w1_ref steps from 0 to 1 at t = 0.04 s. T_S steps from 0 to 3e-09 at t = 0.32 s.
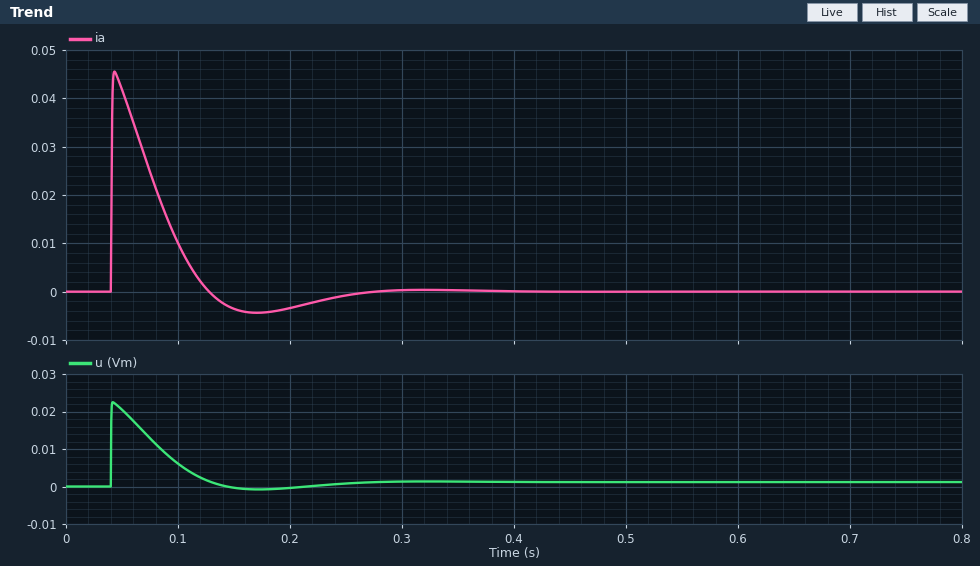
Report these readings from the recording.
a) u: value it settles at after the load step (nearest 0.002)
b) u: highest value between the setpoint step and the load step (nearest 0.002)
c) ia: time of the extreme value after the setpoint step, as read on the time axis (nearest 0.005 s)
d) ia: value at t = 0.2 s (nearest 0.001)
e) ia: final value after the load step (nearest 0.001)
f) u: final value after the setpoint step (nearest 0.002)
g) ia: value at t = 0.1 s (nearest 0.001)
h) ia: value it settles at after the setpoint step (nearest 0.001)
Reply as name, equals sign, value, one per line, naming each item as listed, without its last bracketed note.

u: value it settles at after the load step = 0.002
u: highest value between the setpoint step and the load step = 0.022
ia: time of the extreme value after the setpoint step, as read on the time axis = 0.045 s
ia: value at t = 0.2 s = -0.003
ia: final value after the load step = 0.000
u: final value after the setpoint step = 0.002
ia: value at t = 0.1 s = 0.010
ia: value it settles at after the setpoint step = 0.000
